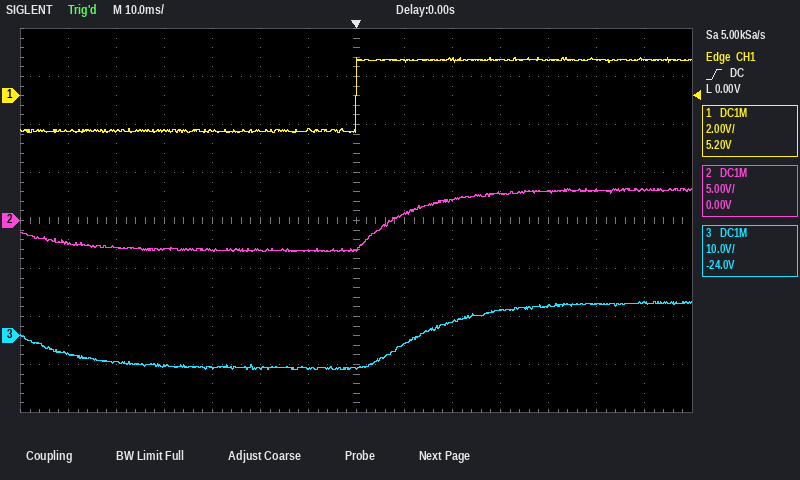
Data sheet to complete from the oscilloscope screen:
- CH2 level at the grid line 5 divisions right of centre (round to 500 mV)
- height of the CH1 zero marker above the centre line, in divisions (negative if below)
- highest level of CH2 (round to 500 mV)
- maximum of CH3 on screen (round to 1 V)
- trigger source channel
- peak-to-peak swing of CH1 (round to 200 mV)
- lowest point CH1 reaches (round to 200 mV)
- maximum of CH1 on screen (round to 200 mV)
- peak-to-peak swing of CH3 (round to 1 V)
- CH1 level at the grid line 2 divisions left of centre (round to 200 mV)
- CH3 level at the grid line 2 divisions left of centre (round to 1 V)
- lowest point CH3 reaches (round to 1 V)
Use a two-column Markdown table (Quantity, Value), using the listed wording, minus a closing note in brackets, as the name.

| Quantity | Value |
|---|---|
| CH2 level at the grid line 5 divisions right of centre | 3.0 V |
| height of the CH1 zero marker above the centre line, in divisions | +2.6 div |
| highest level of CH2 | 3.5 V |
| maximum of CH3 on screen | 7 V |
| trigger source channel | CH1 |
| peak-to-peak swing of CH1 | 3.2 V |
| lowest point CH1 reaches | -1.6 V |
| maximum of CH1 on screen | 1.6 V |
| peak-to-peak swing of CH3 | 14 V |
| CH1 level at the grid line 2 divisions left of centre | -1.4 V |
| CH3 level at the grid line 2 divisions left of centre | -7 V |
| lowest point CH3 reaches | -7 V |
